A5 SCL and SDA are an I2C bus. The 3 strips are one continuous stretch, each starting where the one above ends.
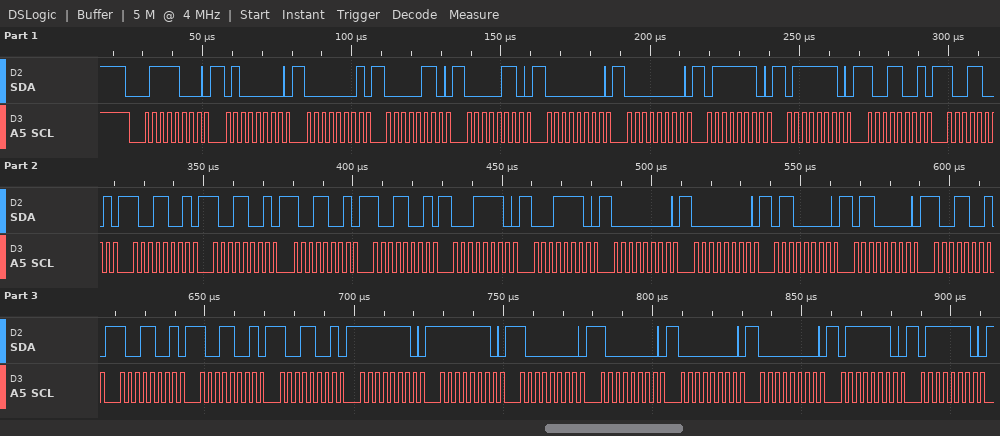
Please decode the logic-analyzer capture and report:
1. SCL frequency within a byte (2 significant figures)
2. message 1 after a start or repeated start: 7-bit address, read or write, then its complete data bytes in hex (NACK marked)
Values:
400 kHz
0x3C write: 40 01 06 06 00 00 7E 7E 99 99 99 99 99 99 1E 1E 00 00 60 60 99 99 99 99 FE FE 80 80 00 00 7E 7E
